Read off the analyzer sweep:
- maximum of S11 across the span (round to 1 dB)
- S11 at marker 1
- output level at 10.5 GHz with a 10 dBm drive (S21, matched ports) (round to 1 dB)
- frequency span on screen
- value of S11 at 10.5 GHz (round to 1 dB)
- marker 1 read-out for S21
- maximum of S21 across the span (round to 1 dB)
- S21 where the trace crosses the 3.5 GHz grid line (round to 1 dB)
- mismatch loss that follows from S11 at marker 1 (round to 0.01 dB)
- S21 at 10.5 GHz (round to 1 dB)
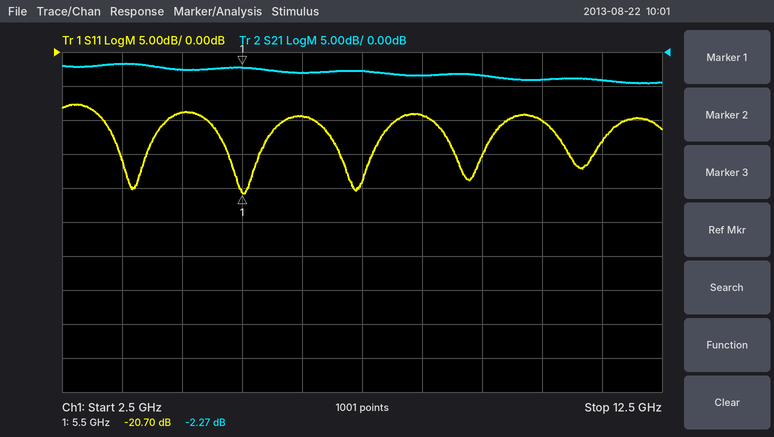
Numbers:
-8 dB
-20.70 dB
6 dBm
10 GHz
-10 dB
-2.27 dB
-2 dB
-2 dB
0.04 dB
-4 dB
